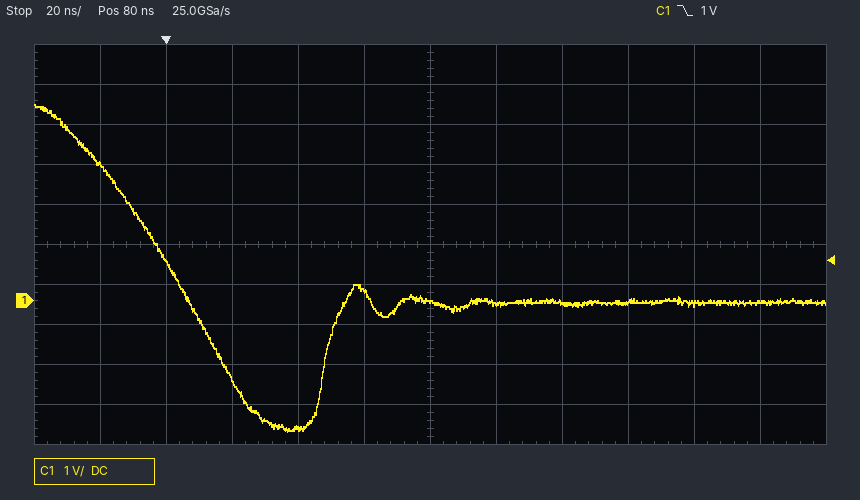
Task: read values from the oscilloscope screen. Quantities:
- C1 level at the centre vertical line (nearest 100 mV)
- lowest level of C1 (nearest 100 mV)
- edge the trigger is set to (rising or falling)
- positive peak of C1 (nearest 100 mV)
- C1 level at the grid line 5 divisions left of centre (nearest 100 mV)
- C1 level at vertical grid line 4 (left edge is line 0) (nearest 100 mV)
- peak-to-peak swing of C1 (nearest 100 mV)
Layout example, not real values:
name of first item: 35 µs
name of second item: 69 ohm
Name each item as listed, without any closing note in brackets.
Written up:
C1 level at the centre vertical line: 0.0 V
lowest level of C1: -3.3 V
edge the trigger is set to: falling
positive peak of C1: 4.9 V
C1 level at the grid line 5 divisions left of centre: 3.4 V
C1 level at vertical grid line 4 (left edge is line 0): -3.2 V
peak-to-peak swing of C1: 8.2 V
